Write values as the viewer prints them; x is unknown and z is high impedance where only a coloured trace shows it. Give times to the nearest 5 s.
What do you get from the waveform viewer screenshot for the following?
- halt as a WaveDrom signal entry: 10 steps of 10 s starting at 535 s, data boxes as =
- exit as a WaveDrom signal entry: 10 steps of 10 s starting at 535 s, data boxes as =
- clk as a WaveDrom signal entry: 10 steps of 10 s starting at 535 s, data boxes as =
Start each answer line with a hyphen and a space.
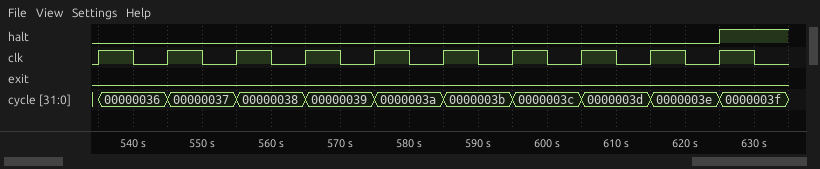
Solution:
- {name: 'halt', wave: '0........1'}
- {name: 'exit', wave: '0.........'}
- {name: 'clk', wave: 'p.........'}
